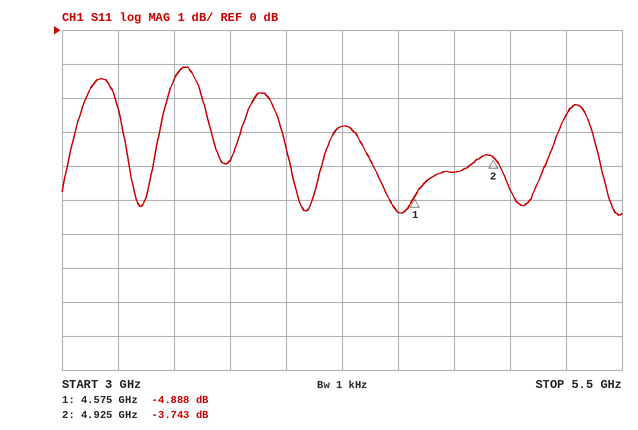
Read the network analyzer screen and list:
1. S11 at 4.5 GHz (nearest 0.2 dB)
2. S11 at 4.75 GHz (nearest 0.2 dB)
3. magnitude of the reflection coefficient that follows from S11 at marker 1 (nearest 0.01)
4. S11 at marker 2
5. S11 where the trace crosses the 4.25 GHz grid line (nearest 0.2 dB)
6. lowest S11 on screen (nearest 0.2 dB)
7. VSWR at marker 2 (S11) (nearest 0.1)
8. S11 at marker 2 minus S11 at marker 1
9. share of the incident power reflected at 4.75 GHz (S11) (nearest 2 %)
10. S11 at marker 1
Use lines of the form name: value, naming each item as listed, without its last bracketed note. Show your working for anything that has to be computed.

S11 at 4.5 GHz: -5.4 dB
S11 at 4.75 GHz: -4.2 dB
magnitude of the reflection coefficient that follows from S11 at marker 1: 10^(-4.888/20) ≈ 0.57
S11 at marker 2: -3.743 dB
S11 where the trace crosses the 4.25 GHz grid line: -2.8 dB
lowest S11 on screen: -5.4 dB
VSWR at marker 2 (S11): (1 + 0.6499)/(1 − 0.6499) ≈ 4.7
S11 at marker 2 minus S11 at marker 1: -3.743 − (-4.888) = 1.145 dB
share of the incident power reflected at 4.75 GHz (S11): 10^(-4.2/10) ≈ 38 %
S11 at marker 1: -4.888 dB
